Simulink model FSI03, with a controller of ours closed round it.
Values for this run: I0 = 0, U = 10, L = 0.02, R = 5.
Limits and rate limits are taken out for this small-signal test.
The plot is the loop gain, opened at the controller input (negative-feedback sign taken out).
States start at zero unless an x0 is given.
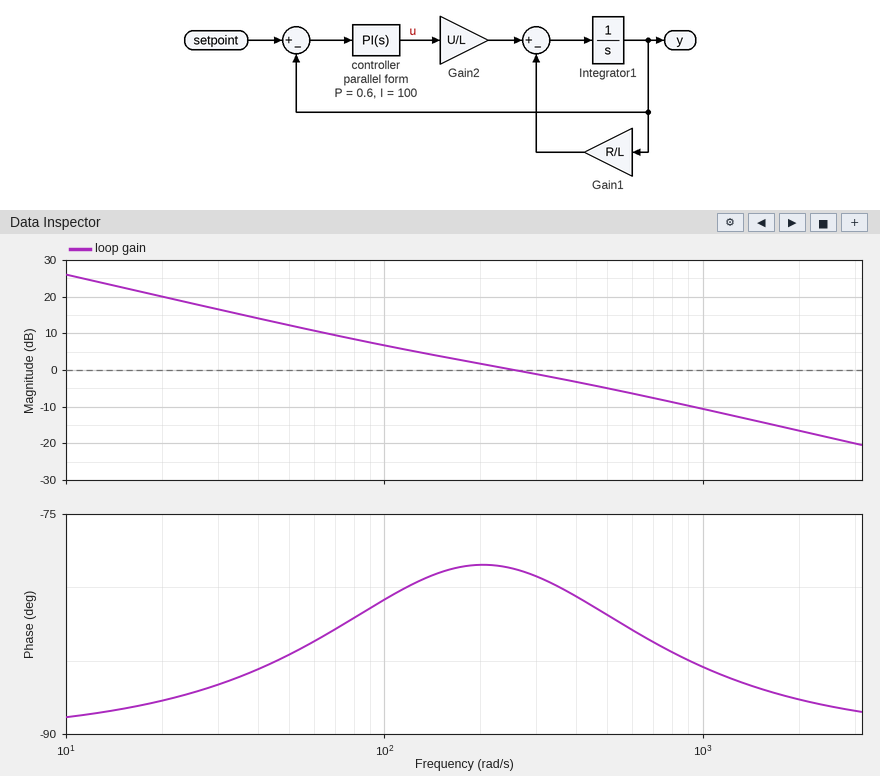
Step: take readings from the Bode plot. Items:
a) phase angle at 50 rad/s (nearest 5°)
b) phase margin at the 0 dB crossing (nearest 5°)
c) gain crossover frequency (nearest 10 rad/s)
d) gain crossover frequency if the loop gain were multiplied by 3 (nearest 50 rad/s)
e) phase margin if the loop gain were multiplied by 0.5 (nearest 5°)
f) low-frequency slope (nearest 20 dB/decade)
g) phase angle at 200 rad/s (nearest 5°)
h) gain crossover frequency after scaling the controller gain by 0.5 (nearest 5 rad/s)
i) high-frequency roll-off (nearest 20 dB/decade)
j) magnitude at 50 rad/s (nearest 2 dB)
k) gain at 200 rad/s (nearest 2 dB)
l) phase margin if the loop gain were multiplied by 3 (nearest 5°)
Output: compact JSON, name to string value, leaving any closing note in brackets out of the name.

{"phase angle at 50 rad/s": "-85°", "phase margin at the 0 dB crossing": "100°", "gain crossover frequency": "260 rad/s", "gain crossover frequency if the loop gain were multiplied by 3": "900 rad/s", "phase margin if the loop gain were multiplied by 0.5": "100°", "low-frequency slope": "-20 dB/decade", "phase angle at 200 rad/s": "-80°", "gain crossover frequency after scaling the controller gain by 0.5": "110 rad/s", "high-frequency roll-off": "-20 dB/decade", "magnitude at 50 rad/s": "12 dB", "gain at 200 rad/s": "2 dB", "phase margin if the loop gain were multiplied by 3": "95°"}
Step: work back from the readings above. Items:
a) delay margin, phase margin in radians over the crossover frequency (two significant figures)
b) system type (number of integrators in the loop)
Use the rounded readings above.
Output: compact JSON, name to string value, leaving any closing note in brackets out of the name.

{"delay margin, phase margin in radians over the crossover frequency": "0.0067 s", "system type": "1"}
